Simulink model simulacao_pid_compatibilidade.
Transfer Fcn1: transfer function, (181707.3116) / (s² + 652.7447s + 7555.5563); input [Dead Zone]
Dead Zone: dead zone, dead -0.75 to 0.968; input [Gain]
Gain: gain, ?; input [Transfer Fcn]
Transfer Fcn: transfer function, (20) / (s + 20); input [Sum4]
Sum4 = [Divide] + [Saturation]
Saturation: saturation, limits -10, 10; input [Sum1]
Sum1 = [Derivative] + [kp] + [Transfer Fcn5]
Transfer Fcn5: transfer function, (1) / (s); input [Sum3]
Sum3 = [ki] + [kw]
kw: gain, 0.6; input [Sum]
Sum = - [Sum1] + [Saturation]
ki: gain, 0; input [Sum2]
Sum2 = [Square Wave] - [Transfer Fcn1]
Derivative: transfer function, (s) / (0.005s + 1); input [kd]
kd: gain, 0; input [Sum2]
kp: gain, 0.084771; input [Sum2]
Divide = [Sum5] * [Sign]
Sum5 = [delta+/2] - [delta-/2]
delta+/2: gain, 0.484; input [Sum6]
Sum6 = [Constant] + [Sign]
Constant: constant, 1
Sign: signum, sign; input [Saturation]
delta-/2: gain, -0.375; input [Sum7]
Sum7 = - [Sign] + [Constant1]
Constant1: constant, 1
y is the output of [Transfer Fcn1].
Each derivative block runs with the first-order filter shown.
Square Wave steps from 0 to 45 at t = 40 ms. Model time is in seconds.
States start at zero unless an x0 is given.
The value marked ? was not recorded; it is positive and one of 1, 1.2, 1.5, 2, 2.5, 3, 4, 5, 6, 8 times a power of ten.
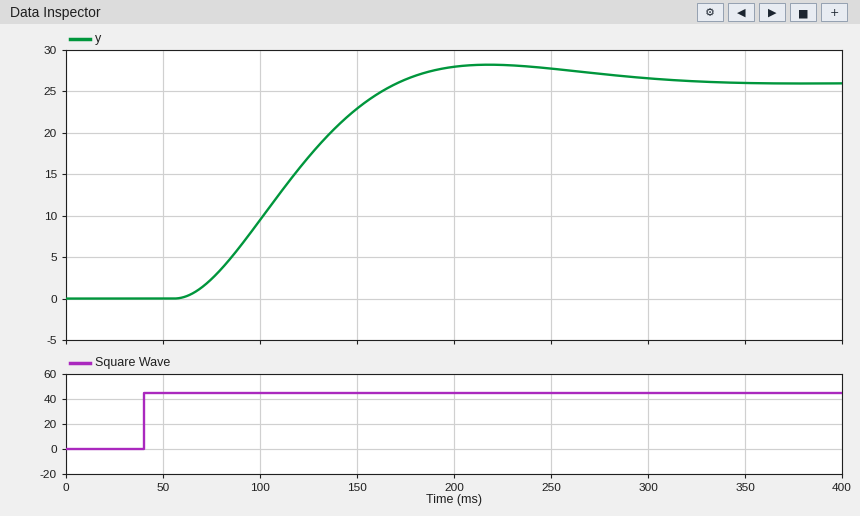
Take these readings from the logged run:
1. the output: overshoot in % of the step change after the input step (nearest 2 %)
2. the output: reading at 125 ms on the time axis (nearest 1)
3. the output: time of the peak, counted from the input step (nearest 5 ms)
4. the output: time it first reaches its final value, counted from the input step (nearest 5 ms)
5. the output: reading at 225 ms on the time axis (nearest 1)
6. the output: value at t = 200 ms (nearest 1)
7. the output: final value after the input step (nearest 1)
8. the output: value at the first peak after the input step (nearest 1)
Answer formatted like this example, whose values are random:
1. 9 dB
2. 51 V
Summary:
1. 8 %
2. 17
3. 180 ms
4. 130 ms
5. 28
6. 28
7. 26
8. 28
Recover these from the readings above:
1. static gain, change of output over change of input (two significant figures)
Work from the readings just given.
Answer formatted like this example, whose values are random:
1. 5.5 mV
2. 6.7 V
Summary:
1. 0.58
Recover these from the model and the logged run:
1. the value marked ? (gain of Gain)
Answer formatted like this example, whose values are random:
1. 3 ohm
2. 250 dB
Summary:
1. 0.8
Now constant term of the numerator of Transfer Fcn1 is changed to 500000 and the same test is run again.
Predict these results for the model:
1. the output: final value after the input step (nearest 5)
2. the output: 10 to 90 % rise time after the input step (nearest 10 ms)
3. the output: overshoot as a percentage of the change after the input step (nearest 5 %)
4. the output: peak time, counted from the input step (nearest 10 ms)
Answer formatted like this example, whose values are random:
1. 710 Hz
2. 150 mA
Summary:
1. 35
2. 40 ms
3. 25 %
4. 110 ms
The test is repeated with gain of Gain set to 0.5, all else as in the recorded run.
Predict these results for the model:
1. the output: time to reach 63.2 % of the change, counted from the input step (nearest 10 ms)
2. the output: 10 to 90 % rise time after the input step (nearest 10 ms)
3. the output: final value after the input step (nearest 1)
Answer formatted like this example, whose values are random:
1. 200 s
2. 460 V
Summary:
1. 110 ms
2. 100 ms
3. 17
